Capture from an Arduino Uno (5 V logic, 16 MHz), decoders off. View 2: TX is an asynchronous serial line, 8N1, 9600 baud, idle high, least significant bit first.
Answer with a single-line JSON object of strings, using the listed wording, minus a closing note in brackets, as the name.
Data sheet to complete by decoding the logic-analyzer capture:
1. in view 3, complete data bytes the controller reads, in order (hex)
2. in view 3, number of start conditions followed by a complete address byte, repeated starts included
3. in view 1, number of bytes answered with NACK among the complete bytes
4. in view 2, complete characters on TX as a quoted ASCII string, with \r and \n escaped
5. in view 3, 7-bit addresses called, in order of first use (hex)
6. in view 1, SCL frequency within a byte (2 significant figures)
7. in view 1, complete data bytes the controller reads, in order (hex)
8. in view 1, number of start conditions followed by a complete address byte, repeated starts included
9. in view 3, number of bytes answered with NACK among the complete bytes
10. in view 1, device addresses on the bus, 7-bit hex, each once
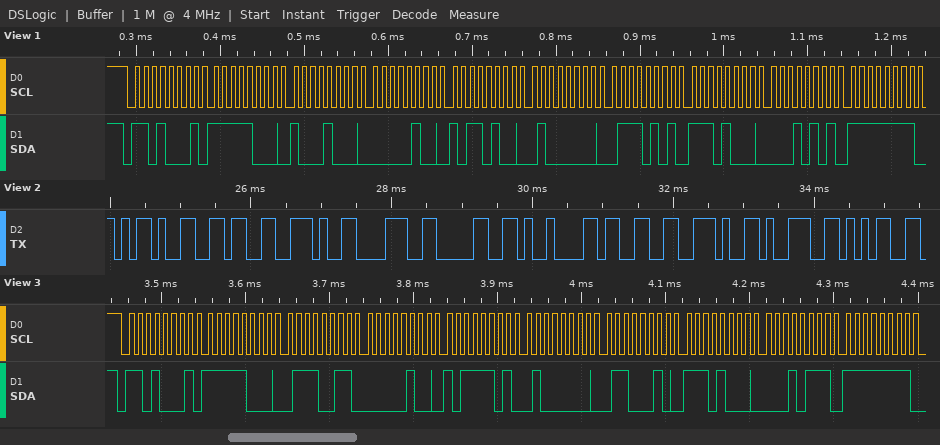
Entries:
{"in view 3, complete data bytes the controller reads, in order": "F8 73 04 BD 40 62 E8 17 FF", "in view 3, number of start conditions followed by a complete address byte, repeated starts included": "1", "in view 1, number of bytes answered with NACK among the complete bytes": "0", "in view 2, complete characters on TX as a quoted ASCII string, with \\r and \\n escaped": "\"-6.80\\t3.95\"", "in view 3, 7-bit addresses called, in order of first use": "0x68", "in view 1, SCL frequency within a byte": "100 kHz", "in view 1, complete data bytes the controller reads, in order": "F8 88 04 B4 40 75 E8 15 FF", "in view 1, number of start conditions followed by a complete address byte, repeated starts included": "1", "in view 3, number of bytes answered with NACK among the complete bytes": "0", "in view 1, device addresses on the bus, 7-bit hex, each once": "0x68"}
